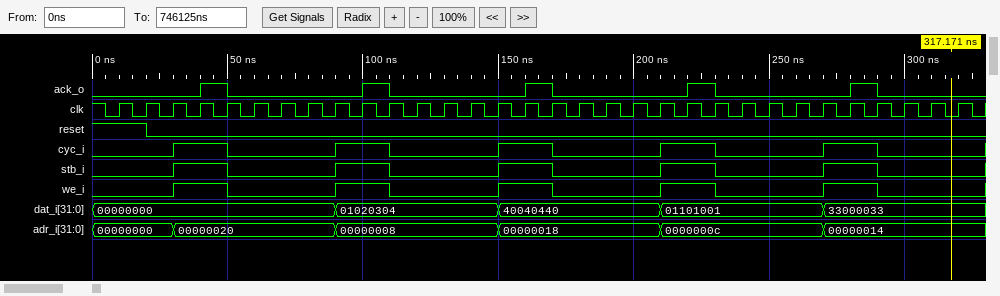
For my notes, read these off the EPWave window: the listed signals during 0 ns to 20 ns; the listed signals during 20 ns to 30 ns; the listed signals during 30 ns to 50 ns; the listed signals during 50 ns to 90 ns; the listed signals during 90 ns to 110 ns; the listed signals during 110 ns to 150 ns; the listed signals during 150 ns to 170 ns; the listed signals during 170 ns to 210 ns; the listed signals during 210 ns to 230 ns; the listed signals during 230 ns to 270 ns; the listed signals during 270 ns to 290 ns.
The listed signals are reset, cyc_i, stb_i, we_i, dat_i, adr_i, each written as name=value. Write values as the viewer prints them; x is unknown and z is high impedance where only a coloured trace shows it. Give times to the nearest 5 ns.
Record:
reset=1, cyc_i=0, stb_i=0, we_i=0, dat_i=00000000, adr_i=00000000
reset=0, cyc_i=0, stb_i=0, we_i=0, dat_i=00000000, adr_i=00000000
reset=0, cyc_i=1, stb_i=1, we_i=1, dat_i=00000000, adr_i=00000020
reset=0, cyc_i=0, stb_i=0, we_i=0, dat_i=00000000, adr_i=00000020
reset=0, cyc_i=1, stb_i=1, we_i=1, dat_i=01020304, adr_i=00000008
reset=0, cyc_i=0, stb_i=0, we_i=0, dat_i=01020304, adr_i=00000008
reset=0, cyc_i=1, stb_i=1, we_i=1, dat_i=40040440, adr_i=00000018
reset=0, cyc_i=0, stb_i=0, we_i=0, dat_i=40040440, adr_i=00000018
reset=0, cyc_i=1, stb_i=1, we_i=1, dat_i=01101001, adr_i=0000000c
reset=0, cyc_i=0, stb_i=0, we_i=0, dat_i=01101001, adr_i=0000000c
reset=0, cyc_i=1, stb_i=1, we_i=1, dat_i=33000033, adr_i=00000014
